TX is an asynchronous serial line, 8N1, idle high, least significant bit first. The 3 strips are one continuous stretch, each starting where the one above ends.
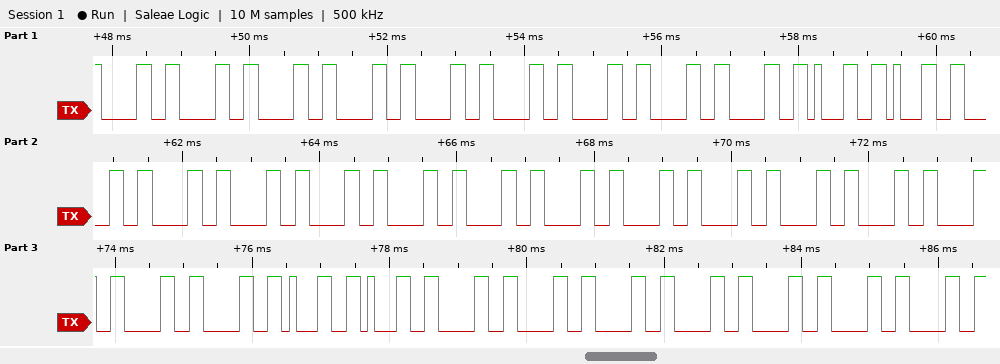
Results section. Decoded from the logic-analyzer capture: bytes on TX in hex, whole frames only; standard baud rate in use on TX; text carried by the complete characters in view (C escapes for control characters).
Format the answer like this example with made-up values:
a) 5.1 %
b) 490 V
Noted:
a) 30 30 30 30 30 30 30 30 30 31 31 30 30 30 30 30 30 30 30 30 30 30 30 30 30 31 31 30 30 30 30 30 30 30
b) 9600 baud
c) "0000000001100000000000000110000000"
